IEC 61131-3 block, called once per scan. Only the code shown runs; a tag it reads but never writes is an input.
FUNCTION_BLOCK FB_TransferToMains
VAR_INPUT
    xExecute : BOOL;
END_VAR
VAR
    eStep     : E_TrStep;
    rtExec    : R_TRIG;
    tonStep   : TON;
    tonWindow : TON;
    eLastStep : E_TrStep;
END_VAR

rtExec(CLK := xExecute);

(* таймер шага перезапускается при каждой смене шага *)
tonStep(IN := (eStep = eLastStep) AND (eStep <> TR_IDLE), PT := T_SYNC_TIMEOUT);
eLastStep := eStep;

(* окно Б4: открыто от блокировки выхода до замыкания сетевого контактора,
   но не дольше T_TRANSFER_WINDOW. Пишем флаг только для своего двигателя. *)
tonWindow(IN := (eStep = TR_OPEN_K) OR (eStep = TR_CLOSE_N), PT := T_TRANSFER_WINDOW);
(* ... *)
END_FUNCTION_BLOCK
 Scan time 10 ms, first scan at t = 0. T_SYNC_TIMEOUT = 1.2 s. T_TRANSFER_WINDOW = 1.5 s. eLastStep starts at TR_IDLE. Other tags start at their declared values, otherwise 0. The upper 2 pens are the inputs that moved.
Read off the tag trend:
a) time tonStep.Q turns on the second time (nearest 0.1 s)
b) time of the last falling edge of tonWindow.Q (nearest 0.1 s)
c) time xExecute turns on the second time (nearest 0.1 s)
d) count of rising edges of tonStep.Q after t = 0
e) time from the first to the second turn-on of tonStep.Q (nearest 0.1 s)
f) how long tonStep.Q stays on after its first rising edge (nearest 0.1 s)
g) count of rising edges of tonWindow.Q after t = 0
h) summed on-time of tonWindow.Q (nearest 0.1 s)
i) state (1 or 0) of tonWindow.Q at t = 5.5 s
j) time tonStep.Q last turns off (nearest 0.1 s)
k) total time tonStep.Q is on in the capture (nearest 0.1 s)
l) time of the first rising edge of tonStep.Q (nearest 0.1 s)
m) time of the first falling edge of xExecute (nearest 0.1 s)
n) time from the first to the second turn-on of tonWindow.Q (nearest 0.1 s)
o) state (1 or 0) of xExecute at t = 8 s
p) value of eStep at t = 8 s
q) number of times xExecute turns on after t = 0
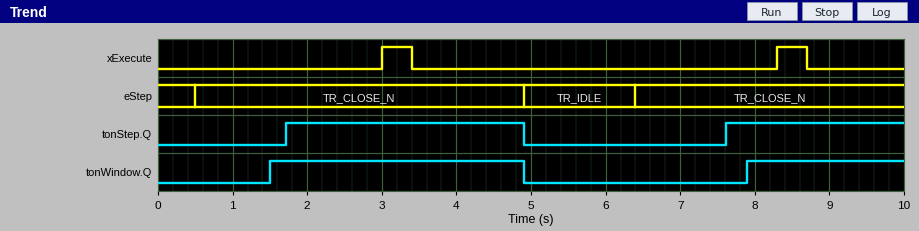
7.6 s
4.9 s
8.3 s
2
5.9 s
3.2 s
2
5.5 s
0
4.9 s
5.6 s
1.7 s
3.4 s
6.4 s
0
TR_CLOSE_N
2
